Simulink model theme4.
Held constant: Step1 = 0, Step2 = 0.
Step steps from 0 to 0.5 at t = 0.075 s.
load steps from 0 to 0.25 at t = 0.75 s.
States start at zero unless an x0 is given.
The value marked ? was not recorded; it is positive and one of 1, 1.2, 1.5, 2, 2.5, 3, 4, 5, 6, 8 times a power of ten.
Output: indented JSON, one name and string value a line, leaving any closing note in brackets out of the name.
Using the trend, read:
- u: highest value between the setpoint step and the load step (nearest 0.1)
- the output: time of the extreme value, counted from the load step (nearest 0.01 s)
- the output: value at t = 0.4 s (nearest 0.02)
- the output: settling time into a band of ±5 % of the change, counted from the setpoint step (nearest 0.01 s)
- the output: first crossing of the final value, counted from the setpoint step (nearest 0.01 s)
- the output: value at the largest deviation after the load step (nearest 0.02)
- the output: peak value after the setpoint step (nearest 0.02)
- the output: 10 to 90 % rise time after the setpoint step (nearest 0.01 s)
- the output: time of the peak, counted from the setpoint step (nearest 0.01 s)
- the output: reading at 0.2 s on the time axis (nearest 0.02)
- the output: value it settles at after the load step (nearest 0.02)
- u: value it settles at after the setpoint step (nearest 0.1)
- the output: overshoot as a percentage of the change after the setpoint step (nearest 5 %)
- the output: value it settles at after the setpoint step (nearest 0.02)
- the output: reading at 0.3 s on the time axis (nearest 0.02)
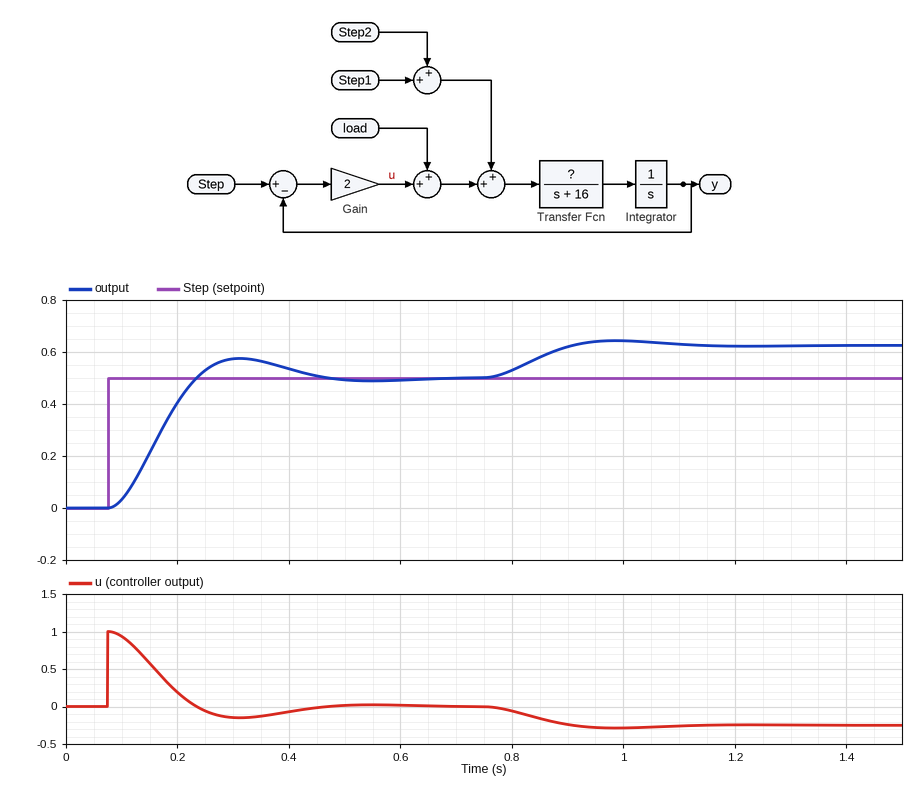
{
  "u: highest value between the setpoint step and the load step": "1.0",
  "the output: time of the extreme value, counted from the load step": "0.24 s",
  "the output: value at t = 0.4 s": "0.54",
  "the output: settling time into a band of ±5 % of the change, counted from the setpoint step": "0.34 s",
  "the output: first crossing of the final value, counted from the setpoint step": "0.16 s",
  "the output: value at the largest deviation after the load step": "0.64",
  "the output: peak value after the setpoint step": "0.58",
  "the output: 10 to 90 % rise time after the setpoint step": "0.11 s",
  "the output: time of the peak, counted from the setpoint step": "0.24 s",
  "the output: reading at 0.2 s on the time axis": "0.40",
  "the output: value it settles at after the load step": "0.62",
  "u: value it settles at after the setpoint step": "0.0",
  "the output: overshoot as a percentage of the change after the setpoint step": "15 %",
  "the output: value it settles at after the setpoint step": "0.50",
  "the output: reading at 0.3 s on the time axis": "0.58"
}
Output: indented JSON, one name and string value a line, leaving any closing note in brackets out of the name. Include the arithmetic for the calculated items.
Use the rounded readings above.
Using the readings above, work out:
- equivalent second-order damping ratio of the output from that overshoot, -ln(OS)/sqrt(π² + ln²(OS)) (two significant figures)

{
  "equivalent second-order damping ratio of the output from that overshoot, -ln(OS)/sqrt(π² + ln²(OS))": "ln(0.15) = -1.897; 1.897 / sqrt(9.870 + 3.599) = 0.52"
}
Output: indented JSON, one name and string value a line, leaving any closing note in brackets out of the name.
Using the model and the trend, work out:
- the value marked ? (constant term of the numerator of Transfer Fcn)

{
  "the value marked ?": "120"
}
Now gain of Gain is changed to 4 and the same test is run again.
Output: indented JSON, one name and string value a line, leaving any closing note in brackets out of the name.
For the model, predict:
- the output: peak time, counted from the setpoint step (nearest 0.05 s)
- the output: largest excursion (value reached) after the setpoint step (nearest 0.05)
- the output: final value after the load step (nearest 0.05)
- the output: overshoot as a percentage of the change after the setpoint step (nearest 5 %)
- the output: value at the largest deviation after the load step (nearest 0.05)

{
  "the output: peak time, counted from the setpoint step": "0.15 s",
  "the output: largest excursion (value reached) after the setpoint step": "0.65",
  "the output: final value after the load step": "0.55",
  "the output: overshoot as a percentage of the change after the setpoint step": "30 %",
  "the output: value at the largest deviation after the load step": "0.60"
}
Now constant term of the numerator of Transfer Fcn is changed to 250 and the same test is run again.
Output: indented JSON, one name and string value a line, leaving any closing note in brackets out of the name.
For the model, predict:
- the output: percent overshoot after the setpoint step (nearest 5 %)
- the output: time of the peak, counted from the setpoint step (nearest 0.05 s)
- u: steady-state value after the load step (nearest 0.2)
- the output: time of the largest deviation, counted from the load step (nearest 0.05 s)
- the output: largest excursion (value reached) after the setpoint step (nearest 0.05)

{
  "the output: percent overshoot after the setpoint step": "30 %",
  "the output: time of the peak, counted from the setpoint step": "0.15 s",
  "u: steady-state value after the load step": "-0.2",
  "the output: time of the largest deviation, counted from the load step": "0.15 s",
  "the output: largest excursion (value reached) after the setpoint step": "0.65"
}
